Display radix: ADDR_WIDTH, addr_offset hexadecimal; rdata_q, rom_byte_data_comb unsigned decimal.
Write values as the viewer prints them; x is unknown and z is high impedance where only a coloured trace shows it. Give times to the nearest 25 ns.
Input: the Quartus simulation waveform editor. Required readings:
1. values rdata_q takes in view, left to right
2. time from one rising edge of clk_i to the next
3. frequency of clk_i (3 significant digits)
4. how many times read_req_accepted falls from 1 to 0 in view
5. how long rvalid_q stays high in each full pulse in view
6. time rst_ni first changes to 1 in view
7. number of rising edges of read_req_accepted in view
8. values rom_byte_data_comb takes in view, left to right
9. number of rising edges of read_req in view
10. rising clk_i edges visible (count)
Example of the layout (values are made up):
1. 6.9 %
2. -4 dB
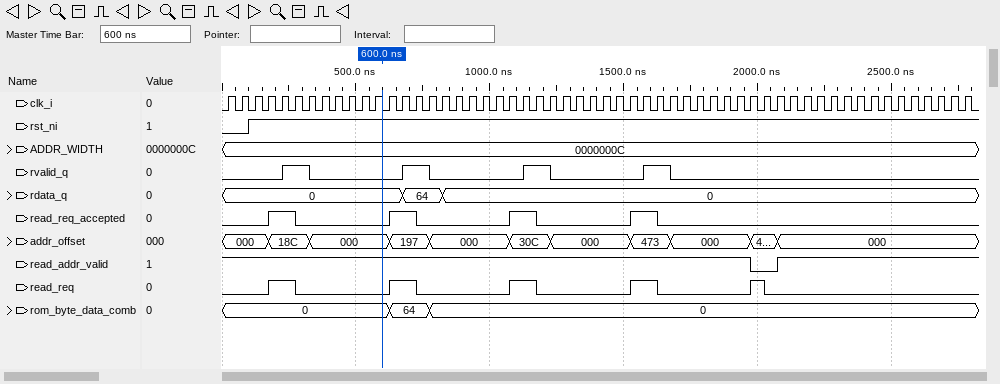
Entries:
1. 0, 64, 0
2. 50 ns
3. 20.0 MHz
4. 4
5. 100 ns, 100 ns, 100 ns, 100 ns
6. 100 ns
7. 4
8. 0, 64, 0
9. 5
10. 56
